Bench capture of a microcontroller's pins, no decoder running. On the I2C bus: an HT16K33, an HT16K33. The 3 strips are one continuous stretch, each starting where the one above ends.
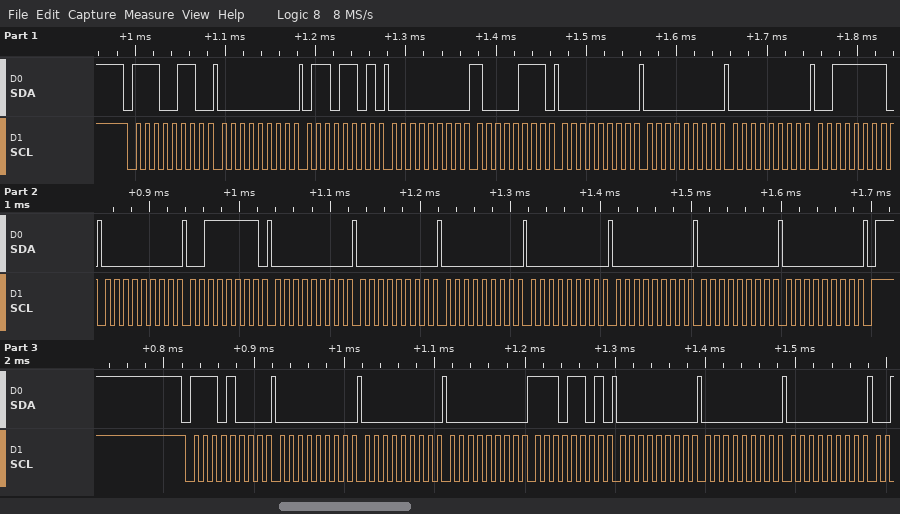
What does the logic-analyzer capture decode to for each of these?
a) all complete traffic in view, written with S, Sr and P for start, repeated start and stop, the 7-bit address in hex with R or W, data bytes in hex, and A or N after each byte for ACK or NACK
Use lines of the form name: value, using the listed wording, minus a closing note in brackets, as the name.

all complete traffic in view, written with S, Sr and P for start, repeated start and stop, the 7-bit address in hex with R or W, data bytes in hex, and A or N after each byte for ACK or NACK: S 73W A 00 A 6D A 00 A 87 A 00 A 00 A 00 A 3F A 00 A 3F A 00 A 00 A 00 A 00 A 00 A 00 A 00 A P S 74W A 00 A 00 A 00 A ED A 00 A 00 A 00 A
